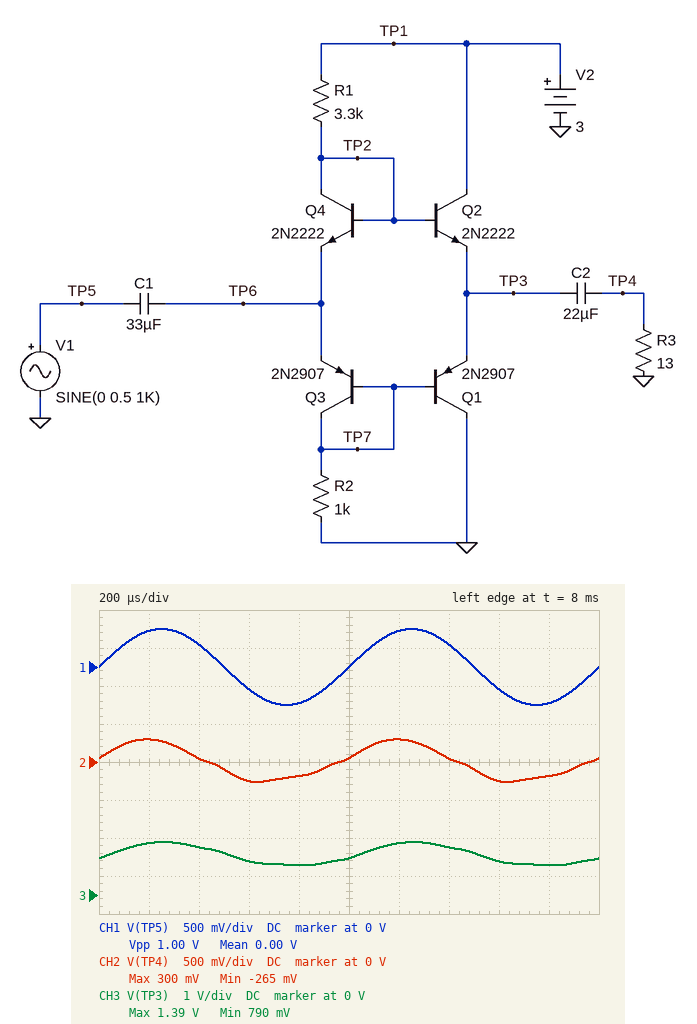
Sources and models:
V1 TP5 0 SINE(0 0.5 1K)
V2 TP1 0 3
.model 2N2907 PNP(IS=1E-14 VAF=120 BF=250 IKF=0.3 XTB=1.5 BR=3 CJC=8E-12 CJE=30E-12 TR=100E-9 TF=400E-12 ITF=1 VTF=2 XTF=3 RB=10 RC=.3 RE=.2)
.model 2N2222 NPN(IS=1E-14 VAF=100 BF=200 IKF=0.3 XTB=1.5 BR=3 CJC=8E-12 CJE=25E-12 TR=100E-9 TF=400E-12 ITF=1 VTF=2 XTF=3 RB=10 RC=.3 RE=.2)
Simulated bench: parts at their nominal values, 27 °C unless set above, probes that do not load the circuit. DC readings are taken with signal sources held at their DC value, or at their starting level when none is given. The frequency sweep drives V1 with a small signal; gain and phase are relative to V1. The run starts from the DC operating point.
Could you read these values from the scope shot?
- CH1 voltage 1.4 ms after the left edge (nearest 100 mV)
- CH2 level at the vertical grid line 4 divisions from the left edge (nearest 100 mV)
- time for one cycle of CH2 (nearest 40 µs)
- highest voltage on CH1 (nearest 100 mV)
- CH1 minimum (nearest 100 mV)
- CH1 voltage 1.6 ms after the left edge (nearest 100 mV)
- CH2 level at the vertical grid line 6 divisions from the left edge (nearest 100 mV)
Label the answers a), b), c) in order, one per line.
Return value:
a) 300 mV
b) -200 mV
c) 1.00 ms
d) 500 mV
e) -500 mV
f) -300 mV
g) 300 mV
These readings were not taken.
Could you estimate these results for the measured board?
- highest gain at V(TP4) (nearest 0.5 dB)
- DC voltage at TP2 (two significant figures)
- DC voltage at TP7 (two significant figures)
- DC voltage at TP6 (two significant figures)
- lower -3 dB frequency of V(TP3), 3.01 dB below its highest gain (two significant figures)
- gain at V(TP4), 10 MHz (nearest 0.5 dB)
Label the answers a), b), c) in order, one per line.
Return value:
a) -6.5 dB
b) 1.7 V
c) 400 mV
d) 1.0 V
e) 5.6 Hz
f) -11.5 dB
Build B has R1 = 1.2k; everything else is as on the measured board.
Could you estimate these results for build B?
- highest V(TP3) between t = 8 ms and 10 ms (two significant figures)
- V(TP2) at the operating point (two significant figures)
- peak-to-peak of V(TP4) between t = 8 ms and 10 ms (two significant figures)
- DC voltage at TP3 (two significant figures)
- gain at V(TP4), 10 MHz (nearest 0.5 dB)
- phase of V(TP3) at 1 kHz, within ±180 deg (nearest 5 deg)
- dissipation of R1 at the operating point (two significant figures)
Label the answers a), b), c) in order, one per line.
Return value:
a) 1.8 V
b) 2.1 V
c) 670 mV
d) 1.4 V
e) -7.5 dB
f) -15 deg
g) 720 µW
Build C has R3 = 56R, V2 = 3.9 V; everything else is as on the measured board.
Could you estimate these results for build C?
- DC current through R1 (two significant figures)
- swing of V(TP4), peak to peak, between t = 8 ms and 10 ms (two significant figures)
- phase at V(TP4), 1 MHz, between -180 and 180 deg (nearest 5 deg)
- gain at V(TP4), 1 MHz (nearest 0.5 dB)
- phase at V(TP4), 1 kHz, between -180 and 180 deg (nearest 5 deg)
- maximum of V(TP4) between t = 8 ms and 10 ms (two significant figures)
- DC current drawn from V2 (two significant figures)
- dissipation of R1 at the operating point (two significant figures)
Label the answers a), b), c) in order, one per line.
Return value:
a) 610 µA
b) 810 mV
c) 0 deg
d) -3.0 dB
e) 5 deg
f) 410 mV
g) 1.2 mA
h) 1.2 mW
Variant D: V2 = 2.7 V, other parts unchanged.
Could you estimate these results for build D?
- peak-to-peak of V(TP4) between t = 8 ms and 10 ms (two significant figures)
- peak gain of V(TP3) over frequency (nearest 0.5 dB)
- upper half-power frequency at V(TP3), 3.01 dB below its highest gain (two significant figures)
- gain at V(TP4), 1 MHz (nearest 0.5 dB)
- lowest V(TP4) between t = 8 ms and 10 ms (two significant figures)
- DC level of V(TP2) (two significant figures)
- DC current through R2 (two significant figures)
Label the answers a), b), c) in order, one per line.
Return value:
a) 510 mV
b) -1.0 dB
c) 160 Hz
d) -12.5 dB
e) -230 mV
f) 1.6 V
g) 340 µA
